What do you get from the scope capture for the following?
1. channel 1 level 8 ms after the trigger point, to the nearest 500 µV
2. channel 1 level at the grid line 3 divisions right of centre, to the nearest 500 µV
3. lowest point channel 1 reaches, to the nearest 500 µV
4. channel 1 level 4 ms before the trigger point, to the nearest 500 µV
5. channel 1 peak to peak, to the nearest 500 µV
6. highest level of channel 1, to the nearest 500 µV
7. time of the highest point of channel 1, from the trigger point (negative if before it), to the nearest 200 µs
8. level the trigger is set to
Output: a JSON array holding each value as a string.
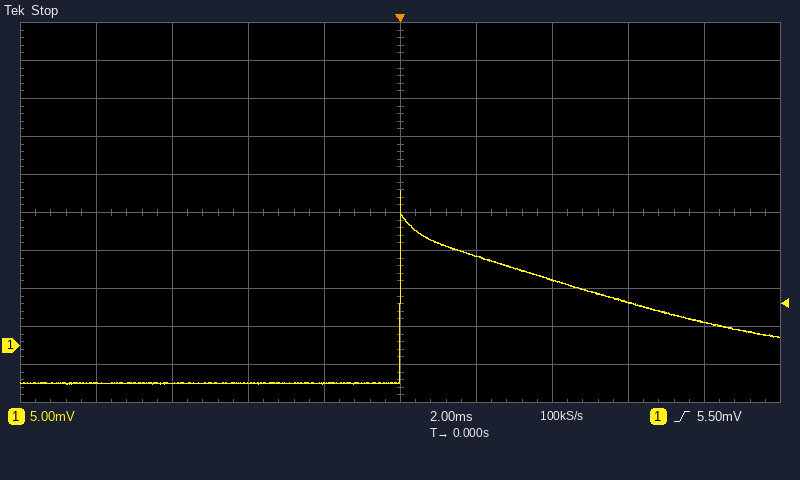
["3.0 mV", "5.5 mV", "-5.0 mV", "-5.0 mV", "25.5 mV", "20.5 mV", "0.0 ms", "5.50 mV"]
